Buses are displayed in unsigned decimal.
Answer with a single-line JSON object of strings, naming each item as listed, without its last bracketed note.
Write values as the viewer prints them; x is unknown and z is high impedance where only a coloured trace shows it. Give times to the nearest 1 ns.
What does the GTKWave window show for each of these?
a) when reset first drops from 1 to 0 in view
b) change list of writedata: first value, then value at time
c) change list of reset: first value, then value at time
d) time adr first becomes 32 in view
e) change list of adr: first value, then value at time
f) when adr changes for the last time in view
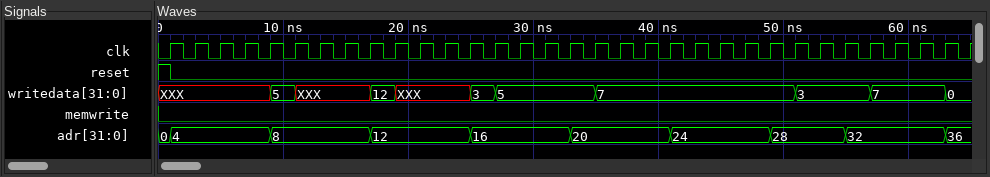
{"when reset first drops from 1 to 0 in view": "1 ns", "change list of writedata: first value, then value at time": "XXX, 5 at 9 ns, XXX at 11 ns, 12 at 17 ns, XXX at 19 ns, 3 at 25 ns, 5 at 27 ns, 7 at 35 ns, 3 at 51 ns, 7 at 57 ns, 0 at 63 ns", "change list of reset: first value, then value at time": "1, 0 at 1 ns", "time adr first becomes 32 in view": "55 ns", "change list of adr: first value, then value at time": "0, 4 at 1 ns, 8 at 9 ns, 12 at 17 ns, 16 at 25 ns, 20 at 33 ns, 24 at 41 ns, 28 at 49 ns, 32 at 55 ns, 36 at 63 ns", "when adr changes for the last time in view": "63 ns"}
